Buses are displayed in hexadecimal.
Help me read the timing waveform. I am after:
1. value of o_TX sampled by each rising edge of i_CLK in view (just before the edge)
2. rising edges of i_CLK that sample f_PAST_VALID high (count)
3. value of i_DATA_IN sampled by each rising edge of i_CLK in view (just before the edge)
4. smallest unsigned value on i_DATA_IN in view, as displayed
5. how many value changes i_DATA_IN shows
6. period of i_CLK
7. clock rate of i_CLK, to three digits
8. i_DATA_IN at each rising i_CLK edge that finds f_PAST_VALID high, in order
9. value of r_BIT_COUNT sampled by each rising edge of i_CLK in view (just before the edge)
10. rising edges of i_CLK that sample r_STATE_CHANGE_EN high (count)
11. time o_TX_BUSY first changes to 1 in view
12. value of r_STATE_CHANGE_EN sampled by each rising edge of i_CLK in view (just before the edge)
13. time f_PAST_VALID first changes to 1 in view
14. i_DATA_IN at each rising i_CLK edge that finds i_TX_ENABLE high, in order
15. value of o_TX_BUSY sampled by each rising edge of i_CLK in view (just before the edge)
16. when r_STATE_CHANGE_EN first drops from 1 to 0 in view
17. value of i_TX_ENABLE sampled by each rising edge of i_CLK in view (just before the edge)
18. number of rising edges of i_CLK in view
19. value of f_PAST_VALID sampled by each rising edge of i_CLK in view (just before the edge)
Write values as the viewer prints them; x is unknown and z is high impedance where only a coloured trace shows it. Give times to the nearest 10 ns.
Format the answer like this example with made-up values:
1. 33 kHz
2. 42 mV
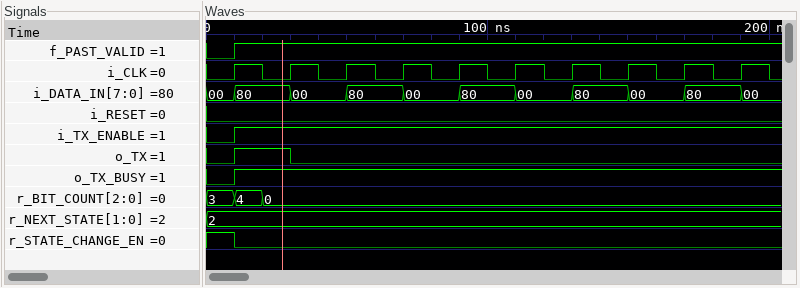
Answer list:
1. 0 1 0 0 0 0 0 0 0 0
2. 9
3. 00, 80, 00, 80, 00, 80, 00, 80, 00, 80
4. 00
5. 10
6. 20 ns
7. 50.0 MHz
8. 80, 00, 80, 00, 80, 00, 80, 00, 80
9. 3, 0, 0, 0, 0, 0, 0, 0, 0, 0
10. 1
11. 10 ns
12. 1 0 0 0 0 0 0 0 0 0
13. 10 ns
14. 80, 00, 80, 00, 80, 00, 80, 00, 80
15. 0 1 1 1 1 1 1 1 1 1
16. 10 ns
17. 0 1 1 1 1 1 1 1 1 1
18. 10
19. 0 1 1 1 1 1 1 1 1 1
